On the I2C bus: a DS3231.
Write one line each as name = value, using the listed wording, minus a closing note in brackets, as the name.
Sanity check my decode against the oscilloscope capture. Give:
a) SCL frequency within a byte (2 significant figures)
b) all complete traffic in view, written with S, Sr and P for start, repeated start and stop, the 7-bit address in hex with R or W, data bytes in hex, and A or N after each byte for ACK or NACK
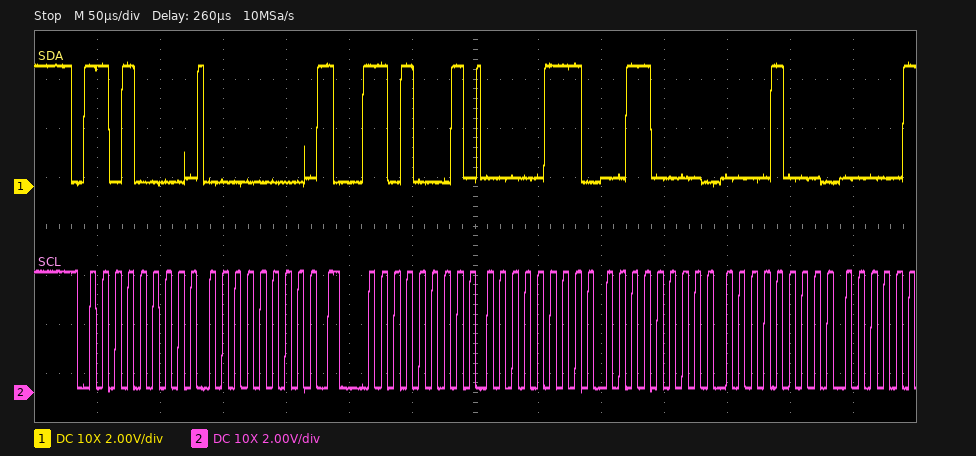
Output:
SCL frequency within a byte = 100 kHz
all complete traffic in view, written with S, Sr and P for start, repeated start and stop, the 7-bit address in hex with R or W, data bytes in hex, and A or N after each byte for ACK or NACK = S 68W A 00 A Sr 68R A 07 A 30 A 08 A
